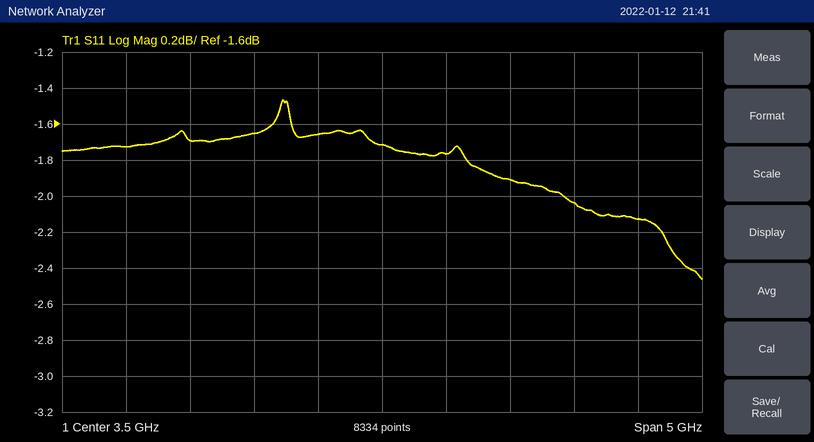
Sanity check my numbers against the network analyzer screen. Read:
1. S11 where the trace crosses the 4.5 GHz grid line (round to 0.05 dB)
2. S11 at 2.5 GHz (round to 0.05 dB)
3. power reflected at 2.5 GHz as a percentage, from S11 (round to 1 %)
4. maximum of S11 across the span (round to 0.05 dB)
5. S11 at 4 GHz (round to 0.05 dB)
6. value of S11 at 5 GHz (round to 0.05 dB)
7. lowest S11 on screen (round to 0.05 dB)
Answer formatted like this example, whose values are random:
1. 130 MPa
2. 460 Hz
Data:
1. -1.90 dB
2. -1.65 dB
3. 68 %
4. -1.45 dB
5. -1.75 dB
6. -2.05 dB
7. -2.45 dB
